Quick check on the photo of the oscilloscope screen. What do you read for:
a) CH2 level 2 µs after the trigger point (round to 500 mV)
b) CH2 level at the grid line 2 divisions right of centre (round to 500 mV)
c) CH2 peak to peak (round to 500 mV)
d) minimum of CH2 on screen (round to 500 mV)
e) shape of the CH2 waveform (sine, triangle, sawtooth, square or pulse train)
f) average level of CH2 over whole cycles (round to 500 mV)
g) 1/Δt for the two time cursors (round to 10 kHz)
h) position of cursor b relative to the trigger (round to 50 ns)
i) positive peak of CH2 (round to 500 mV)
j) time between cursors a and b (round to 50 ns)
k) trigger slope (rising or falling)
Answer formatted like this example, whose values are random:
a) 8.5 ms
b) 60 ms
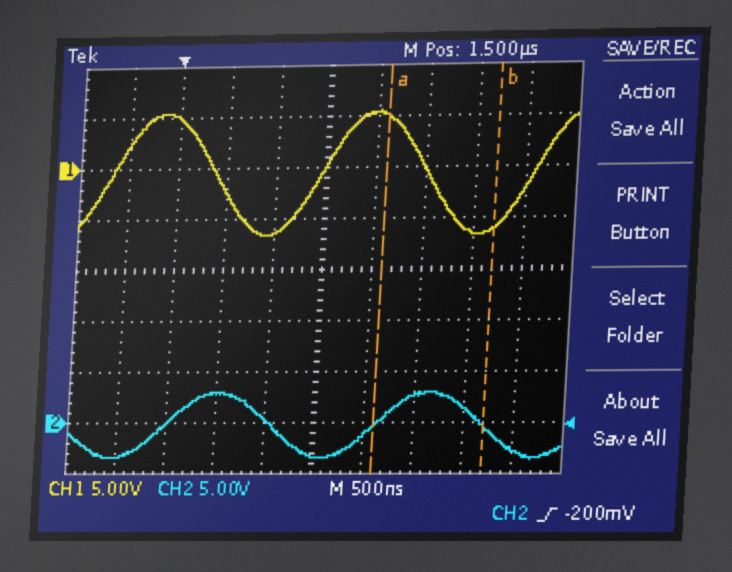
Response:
a) -1.5 V
b) 2.5 V
c) 6.5 V
d) -3.5 V
e) sine
f) 0.0 V
g) 910 kHz
h) +3.20 µs
i) 3.0 V
j) 1.10 µs
k) rising
